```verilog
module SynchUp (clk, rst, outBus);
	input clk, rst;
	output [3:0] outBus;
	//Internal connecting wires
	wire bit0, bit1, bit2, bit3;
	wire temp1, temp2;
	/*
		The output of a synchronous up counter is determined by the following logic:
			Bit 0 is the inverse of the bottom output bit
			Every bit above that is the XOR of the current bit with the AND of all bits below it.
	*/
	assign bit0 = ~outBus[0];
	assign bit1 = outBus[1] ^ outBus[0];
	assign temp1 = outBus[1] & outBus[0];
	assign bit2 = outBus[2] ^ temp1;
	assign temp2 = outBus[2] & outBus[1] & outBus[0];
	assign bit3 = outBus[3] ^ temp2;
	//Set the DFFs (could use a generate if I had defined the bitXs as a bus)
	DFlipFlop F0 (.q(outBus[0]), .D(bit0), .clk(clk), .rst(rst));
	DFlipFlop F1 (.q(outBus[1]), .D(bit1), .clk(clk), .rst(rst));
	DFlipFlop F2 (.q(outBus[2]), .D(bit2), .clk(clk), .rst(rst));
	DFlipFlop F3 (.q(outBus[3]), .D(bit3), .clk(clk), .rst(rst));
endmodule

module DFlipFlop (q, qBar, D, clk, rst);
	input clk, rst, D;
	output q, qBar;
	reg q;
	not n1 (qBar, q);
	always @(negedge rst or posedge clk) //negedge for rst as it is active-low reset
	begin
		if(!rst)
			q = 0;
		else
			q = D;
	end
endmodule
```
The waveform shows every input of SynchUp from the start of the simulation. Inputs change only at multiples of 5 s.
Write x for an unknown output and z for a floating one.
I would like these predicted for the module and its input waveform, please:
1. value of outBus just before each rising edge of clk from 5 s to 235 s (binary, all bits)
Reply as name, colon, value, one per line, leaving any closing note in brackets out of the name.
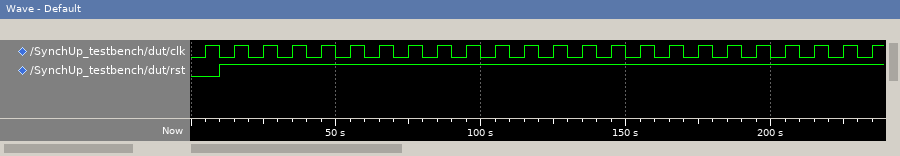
value of outBus just before each rising edge of clk from 5 s to 235 s: 0000, 0000, 0001, 0010, 0011, 0100, 0101, 0110, 0111, 1000, 1001, 1010, 1011, 1100, 1101, 1110, 1111, 0000, 0001, 0010, 0011, 0100, 0101, 0110
